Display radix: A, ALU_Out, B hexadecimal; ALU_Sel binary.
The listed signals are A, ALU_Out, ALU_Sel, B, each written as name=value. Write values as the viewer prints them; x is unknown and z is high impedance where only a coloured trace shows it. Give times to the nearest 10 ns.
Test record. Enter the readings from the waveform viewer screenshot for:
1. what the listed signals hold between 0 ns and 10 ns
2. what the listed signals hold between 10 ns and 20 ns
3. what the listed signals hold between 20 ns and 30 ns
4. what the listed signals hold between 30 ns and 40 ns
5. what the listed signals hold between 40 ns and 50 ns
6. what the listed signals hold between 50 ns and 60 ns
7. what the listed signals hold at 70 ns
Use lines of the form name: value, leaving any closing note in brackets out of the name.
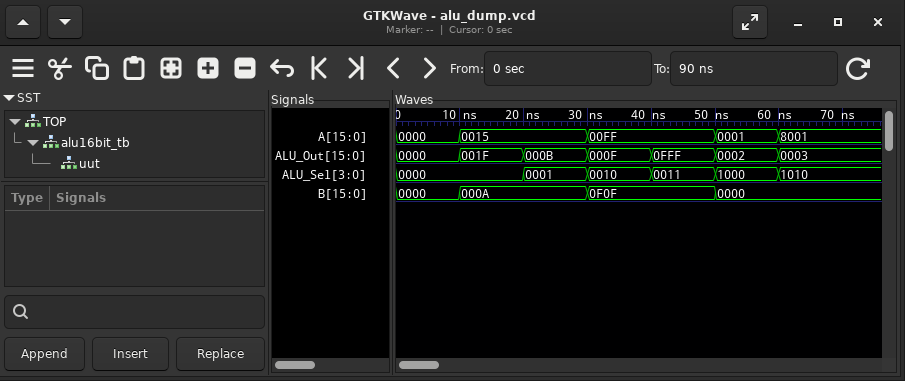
what the listed signals hold between 0 ns and 10 ns: A=0000, ALU_Out=0000, ALU_Sel=0000, B=0000
what the listed signals hold between 10 ns and 20 ns: A=0015, ALU_Out=001F, ALU_Sel=0000, B=000A
what the listed signals hold between 20 ns and 30 ns: A=0015, ALU_Out=000B, ALU_Sel=0001, B=000A
what the listed signals hold between 30 ns and 40 ns: A=00FF, ALU_Out=000F, ALU_Sel=0010, B=0F0F
what the listed signals hold between 40 ns and 50 ns: A=00FF, ALU_Out=0FFF, ALU_Sel=0011, B=0F0F
what the listed signals hold between 50 ns and 60 ns: A=0001, ALU_Out=0002, ALU_Sel=1000, B=0000
what the listed signals hold at 70 ns: A=8001, ALU_Out=0003, ALU_Sel=1010, B=0000
